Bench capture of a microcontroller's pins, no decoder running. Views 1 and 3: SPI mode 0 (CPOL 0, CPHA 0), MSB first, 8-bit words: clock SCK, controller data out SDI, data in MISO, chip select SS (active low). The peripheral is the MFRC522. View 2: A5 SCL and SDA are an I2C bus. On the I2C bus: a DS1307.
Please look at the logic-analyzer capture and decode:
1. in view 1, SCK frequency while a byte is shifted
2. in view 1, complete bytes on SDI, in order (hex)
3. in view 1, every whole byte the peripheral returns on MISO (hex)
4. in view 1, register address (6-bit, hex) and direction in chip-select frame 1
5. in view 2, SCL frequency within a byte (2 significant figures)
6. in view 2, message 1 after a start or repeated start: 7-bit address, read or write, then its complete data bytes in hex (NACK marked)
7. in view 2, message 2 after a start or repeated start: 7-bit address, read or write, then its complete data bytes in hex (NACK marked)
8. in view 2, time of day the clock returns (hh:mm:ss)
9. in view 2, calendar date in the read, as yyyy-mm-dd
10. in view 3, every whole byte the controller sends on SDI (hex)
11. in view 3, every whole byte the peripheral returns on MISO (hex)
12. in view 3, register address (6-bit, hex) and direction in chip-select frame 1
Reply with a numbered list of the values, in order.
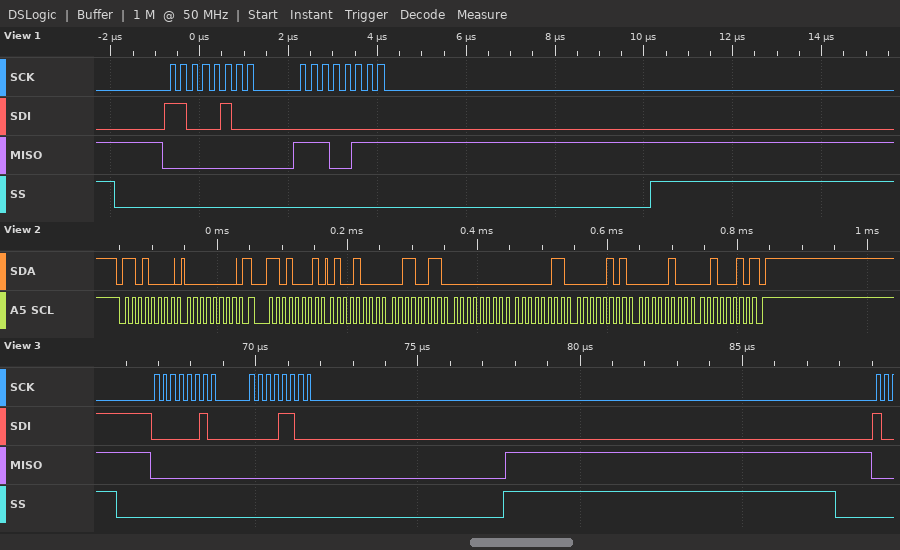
1. 4 MHz
2. C4 00
3. 00 E7
4. 0x22 read
5. 100 kHz
6. 0x68 write: 00
7. 0x68 read: 48 33 00 03 05 04 22 NACK
8. 00:33:48
9. 2022-04-05
10. 0x02 0x0C
11. 0x00 0x00
12. 0x01 write
